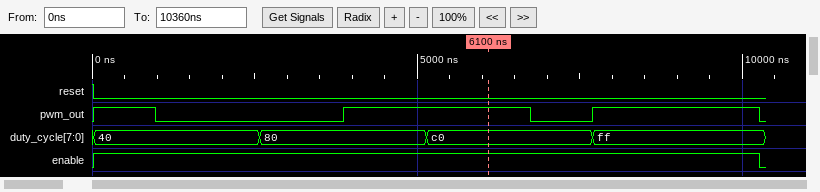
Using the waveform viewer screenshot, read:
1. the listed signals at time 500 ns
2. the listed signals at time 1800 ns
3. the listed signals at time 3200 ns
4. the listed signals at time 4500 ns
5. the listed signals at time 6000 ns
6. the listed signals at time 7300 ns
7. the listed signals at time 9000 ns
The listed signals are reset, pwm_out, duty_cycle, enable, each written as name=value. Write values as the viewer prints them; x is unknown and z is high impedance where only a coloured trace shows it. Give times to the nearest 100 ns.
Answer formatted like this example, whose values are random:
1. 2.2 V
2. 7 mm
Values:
1. reset=0, pwm_out=1, duty_cycle=40, enable=1
2. reset=0, pwm_out=0, duty_cycle=40, enable=1
3. reset=0, pwm_out=0, duty_cycle=80, enable=1
4. reset=0, pwm_out=1, duty_cycle=80, enable=1
5. reset=0, pwm_out=1, duty_cycle=c0, enable=1
6. reset=0, pwm_out=0, duty_cycle=c0, enable=1
7. reset=0, pwm_out=1, duty_cycle=ff, enable=1
